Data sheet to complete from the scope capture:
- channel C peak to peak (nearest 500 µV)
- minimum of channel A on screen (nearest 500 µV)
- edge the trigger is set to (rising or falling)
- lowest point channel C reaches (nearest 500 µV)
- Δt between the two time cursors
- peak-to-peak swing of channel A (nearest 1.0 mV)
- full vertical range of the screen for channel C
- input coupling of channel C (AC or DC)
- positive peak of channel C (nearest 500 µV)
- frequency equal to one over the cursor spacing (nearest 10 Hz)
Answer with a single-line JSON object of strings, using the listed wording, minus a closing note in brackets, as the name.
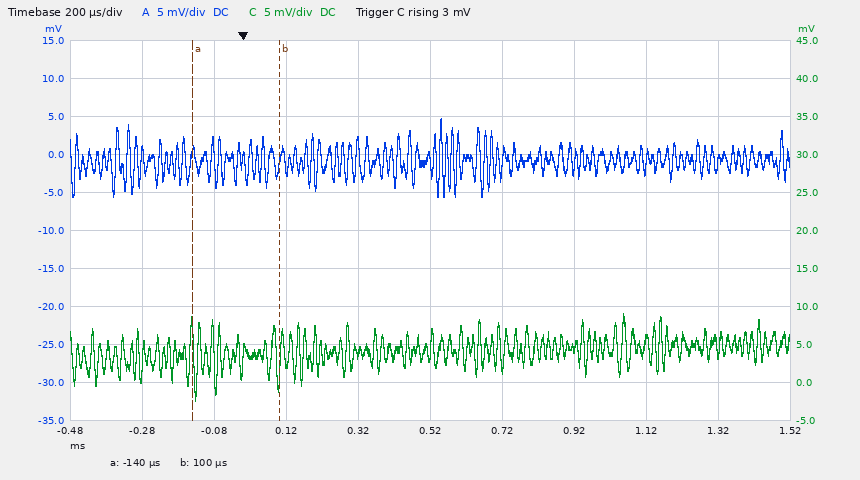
{"channel C peak to peak": "11.5 mV", "minimum of channel A on screen": "-5.5 mV", "edge the trigger is set to": "rising", "lowest point channel C reaches": "-2.5 mV", "Δt between the two time cursors": "240 µs", "peak-to-peak swing of channel A": "10.0 mV", "full vertical range of the screen for channel C": "50 mV", "input coupling of channel C": "DC", "positive peak of channel C": "9.0 mV", "frequency equal to one over the cursor spacing": "4.17 kHz"}
